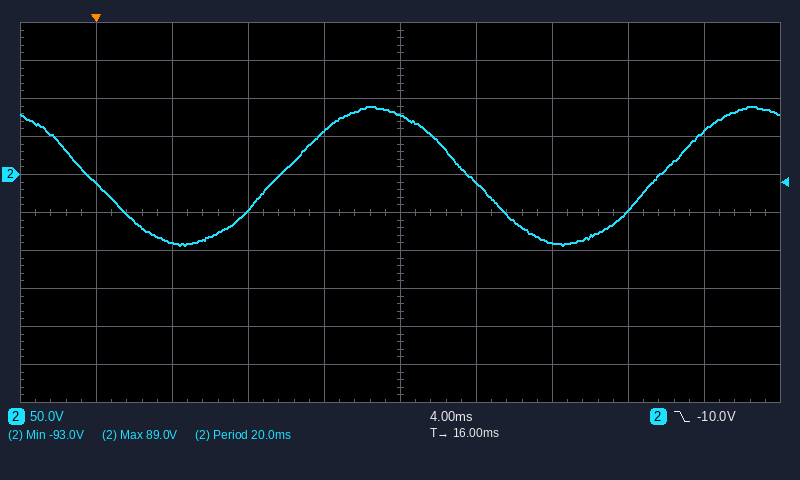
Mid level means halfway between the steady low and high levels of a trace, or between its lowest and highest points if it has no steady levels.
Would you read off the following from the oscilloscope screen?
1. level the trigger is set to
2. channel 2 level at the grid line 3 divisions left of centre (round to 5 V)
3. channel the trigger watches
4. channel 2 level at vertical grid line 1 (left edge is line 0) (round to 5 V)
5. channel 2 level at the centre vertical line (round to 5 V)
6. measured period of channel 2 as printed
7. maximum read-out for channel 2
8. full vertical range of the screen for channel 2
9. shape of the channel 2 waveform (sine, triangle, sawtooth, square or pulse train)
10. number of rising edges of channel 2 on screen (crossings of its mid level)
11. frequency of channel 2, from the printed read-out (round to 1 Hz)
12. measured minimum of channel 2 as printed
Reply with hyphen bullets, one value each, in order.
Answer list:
- -10.0 V
- -90 V
- channel 2
- -10 V
- 80 V
- 20.0 ms
- 89.0 V
- 500 V
- sine
- 2
- 50 Hz
- -93.0 V
